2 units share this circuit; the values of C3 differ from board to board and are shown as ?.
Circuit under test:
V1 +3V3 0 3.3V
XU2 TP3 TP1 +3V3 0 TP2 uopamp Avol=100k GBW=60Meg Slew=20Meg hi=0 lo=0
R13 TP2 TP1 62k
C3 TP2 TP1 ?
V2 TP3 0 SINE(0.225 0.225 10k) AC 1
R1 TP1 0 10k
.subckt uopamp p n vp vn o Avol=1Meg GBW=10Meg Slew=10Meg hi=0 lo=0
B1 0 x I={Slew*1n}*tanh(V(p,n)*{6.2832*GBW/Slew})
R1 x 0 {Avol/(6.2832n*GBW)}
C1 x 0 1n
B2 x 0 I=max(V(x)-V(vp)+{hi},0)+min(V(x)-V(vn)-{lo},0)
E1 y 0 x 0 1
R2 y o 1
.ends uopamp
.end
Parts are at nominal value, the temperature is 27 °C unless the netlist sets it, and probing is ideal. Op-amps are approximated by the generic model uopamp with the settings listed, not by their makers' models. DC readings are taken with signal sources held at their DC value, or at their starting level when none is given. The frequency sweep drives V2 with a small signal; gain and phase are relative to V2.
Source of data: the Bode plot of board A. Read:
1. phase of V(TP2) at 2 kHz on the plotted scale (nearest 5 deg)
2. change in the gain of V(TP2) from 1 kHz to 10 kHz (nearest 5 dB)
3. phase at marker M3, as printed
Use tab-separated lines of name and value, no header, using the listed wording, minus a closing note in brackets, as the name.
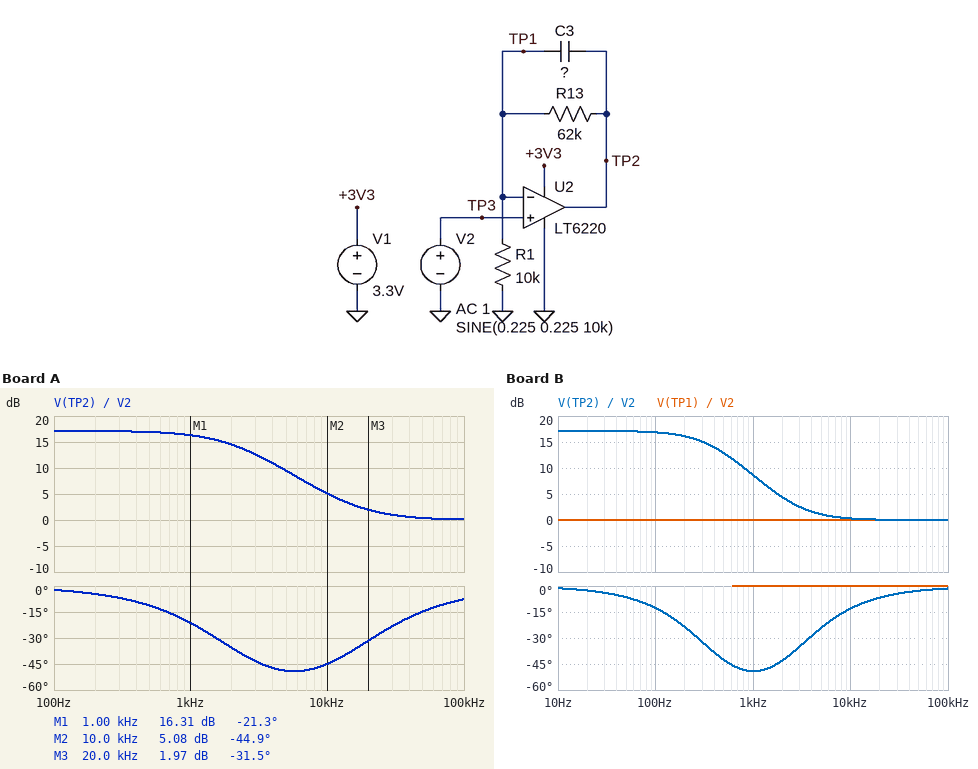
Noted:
phase of V(TP2) at 2 kHz on the plotted scale	-35 deg
change in the gain of V(TP2) from 1 kHz to 10 kHz	-10 dB
phase at marker M3, as printed	-31.5 deg
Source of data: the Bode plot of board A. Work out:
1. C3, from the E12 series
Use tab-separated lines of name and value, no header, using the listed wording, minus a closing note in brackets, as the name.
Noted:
C3, from the E12 series	1.2 nF
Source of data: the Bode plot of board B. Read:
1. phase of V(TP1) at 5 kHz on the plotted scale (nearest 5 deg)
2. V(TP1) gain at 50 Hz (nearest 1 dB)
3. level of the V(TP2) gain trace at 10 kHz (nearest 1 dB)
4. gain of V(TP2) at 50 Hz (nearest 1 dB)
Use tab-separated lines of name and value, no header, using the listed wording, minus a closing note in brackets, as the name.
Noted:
phase of V(TP1) at 5 kHz on the plotted scale	0 deg
V(TP1) gain at 50 Hz	0 dB
level of the V(TP2) gain trace at 10 kHz	0 dB
gain of V(TP2) at 50 Hz	17 dB
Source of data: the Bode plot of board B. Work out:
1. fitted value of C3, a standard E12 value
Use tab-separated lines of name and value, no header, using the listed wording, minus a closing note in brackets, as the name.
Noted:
fitted value of C3, a standard E12 value	6.8 nF
